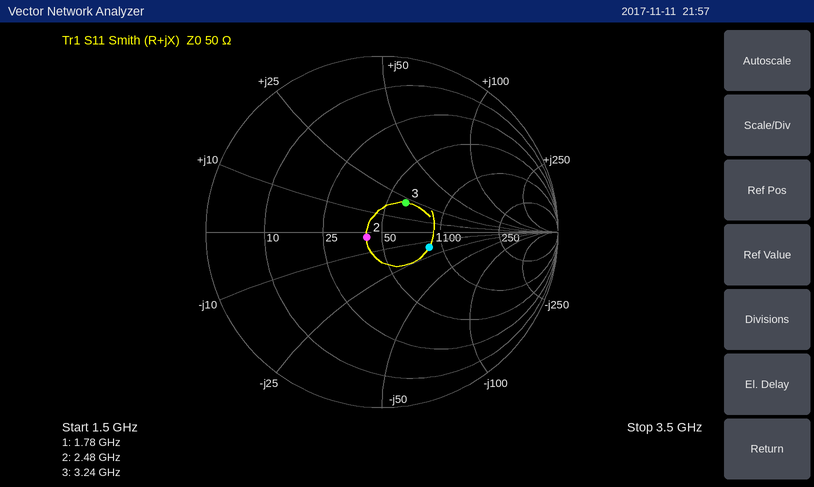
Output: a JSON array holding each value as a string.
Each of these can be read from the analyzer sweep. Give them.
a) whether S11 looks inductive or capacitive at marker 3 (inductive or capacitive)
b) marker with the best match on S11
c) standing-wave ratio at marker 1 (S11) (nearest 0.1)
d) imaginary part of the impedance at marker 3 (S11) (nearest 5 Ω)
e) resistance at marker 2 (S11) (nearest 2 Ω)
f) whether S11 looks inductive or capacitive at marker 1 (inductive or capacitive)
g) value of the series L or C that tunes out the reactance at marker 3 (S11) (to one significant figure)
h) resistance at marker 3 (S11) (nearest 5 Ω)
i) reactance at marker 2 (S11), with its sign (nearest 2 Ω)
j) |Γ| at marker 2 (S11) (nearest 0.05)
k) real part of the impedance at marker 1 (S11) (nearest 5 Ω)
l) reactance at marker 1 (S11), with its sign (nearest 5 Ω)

["inductive", "marker 2", "1.8", "+20 Ω", "42 Ω", "capacitive", "2 pF", "60 Ω", "-2 Ω", "0.10", "85 Ω", "-15 Ω"]
